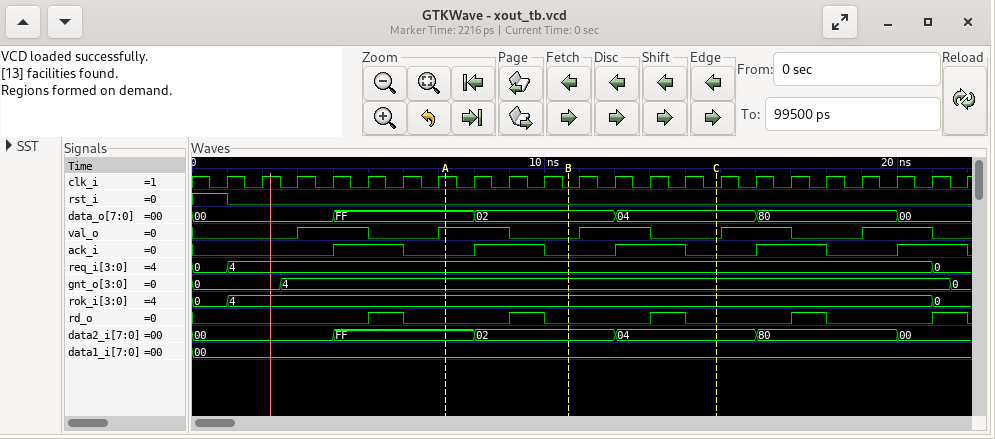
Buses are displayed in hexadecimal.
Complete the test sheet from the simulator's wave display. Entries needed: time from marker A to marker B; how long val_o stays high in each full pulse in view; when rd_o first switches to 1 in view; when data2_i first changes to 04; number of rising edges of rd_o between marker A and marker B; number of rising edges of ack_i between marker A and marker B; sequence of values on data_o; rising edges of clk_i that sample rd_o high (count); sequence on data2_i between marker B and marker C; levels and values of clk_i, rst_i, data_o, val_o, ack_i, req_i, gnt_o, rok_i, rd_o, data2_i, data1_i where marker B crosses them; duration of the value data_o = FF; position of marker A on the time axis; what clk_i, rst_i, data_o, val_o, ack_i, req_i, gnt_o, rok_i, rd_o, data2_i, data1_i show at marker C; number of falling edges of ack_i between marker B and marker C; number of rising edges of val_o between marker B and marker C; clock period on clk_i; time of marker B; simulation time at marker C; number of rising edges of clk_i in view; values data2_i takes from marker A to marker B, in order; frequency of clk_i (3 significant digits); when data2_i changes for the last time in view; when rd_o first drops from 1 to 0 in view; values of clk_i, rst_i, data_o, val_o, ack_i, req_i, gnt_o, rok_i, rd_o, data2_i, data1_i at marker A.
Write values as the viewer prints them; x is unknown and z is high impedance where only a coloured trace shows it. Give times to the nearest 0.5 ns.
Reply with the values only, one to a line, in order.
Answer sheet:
3.5 ns
2 ns, 2 ns, 2 ns, 2 ns, 2 ns
5 ns
12 ns
1
1
00, FF, 02, 04, 80, 00
5
02, 04
clk_i=0, rst_i=0, data_o=02, val_o=0, ack_i=0, req_i=4, gnt_o=4, rok_i=4, rd_o=0, data2_i=02, data1_i=00
4 ns
7 ns
clk_i=0, rst_i=0, data_o=04, val_o=0, ack_i=0, req_i=4, gnt_o=4, rok_i=4, rd_o=0, data2_i=04, data1_i=00
1
1
1 ns
10.5 ns
15 ns
22
FF, 02
1.00 GHz
20 ns
6 ns
clk_i=1, rst_i=0, data_o=FF, val_o=1, ack_i=0, req_i=4, gnt_o=4, rok_i=4, rd_o=0, data2_i=FF, data1_i=00
